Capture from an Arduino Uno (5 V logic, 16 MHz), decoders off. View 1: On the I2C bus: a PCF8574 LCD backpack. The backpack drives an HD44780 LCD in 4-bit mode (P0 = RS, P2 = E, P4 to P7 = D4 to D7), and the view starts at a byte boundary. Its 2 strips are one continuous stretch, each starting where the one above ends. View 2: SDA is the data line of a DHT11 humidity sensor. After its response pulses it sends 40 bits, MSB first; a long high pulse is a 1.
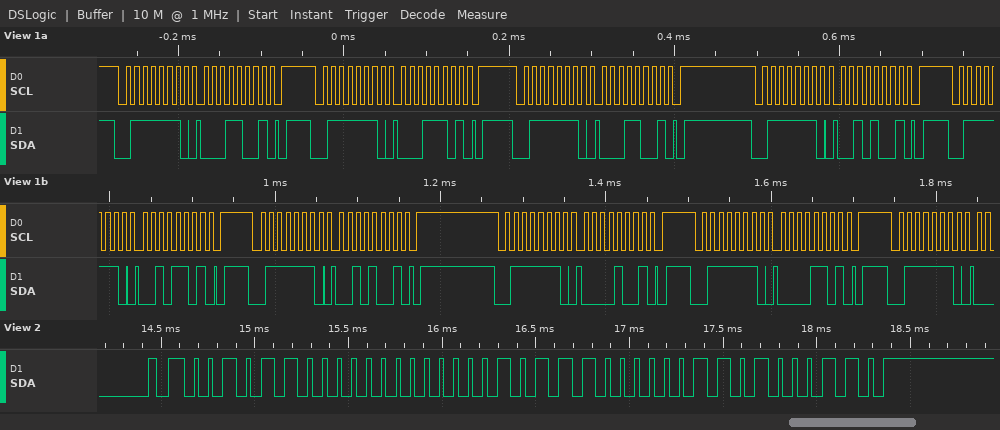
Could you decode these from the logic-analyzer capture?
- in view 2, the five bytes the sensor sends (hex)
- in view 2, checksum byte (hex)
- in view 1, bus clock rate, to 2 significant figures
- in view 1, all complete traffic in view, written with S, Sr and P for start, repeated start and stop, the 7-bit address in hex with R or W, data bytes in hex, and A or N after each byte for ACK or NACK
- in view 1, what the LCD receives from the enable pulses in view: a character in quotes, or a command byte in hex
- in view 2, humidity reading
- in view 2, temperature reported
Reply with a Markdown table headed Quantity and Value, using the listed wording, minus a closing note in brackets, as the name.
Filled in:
| Quantity | Value |
|---|---|
| in view 2, the five bytes the sensor sends | 2C 00 17 03 46 |
| in view 2, checksum byte | 0x46 |
| in view 1, bus clock rate, to 2 significant figures | 100 kHz |
| in view 1, all complete traffic in view, written with S, Sr and P for start, repeated start and stop, the 7-bit address in hex with R or W, data bytes in hex, and A or N after each byte for ACK or NACK | S 3FW A 19 A P S 3FW A 1D A P S 3FW A 19 A P S 3FW A 29 A P S 3FW A 2D A P S 3FW A 29 A P S 3FW A 09 A P S 3FW A 0D A P S 3FW A |
| in view 1, what the LCD receives from the enable pulses in view: a character in quotes, or a command byte in hex | data 0x12 |
| in view 2, humidity reading | 44 % |
| in view 2, temperature reported | 23.3 °C |
